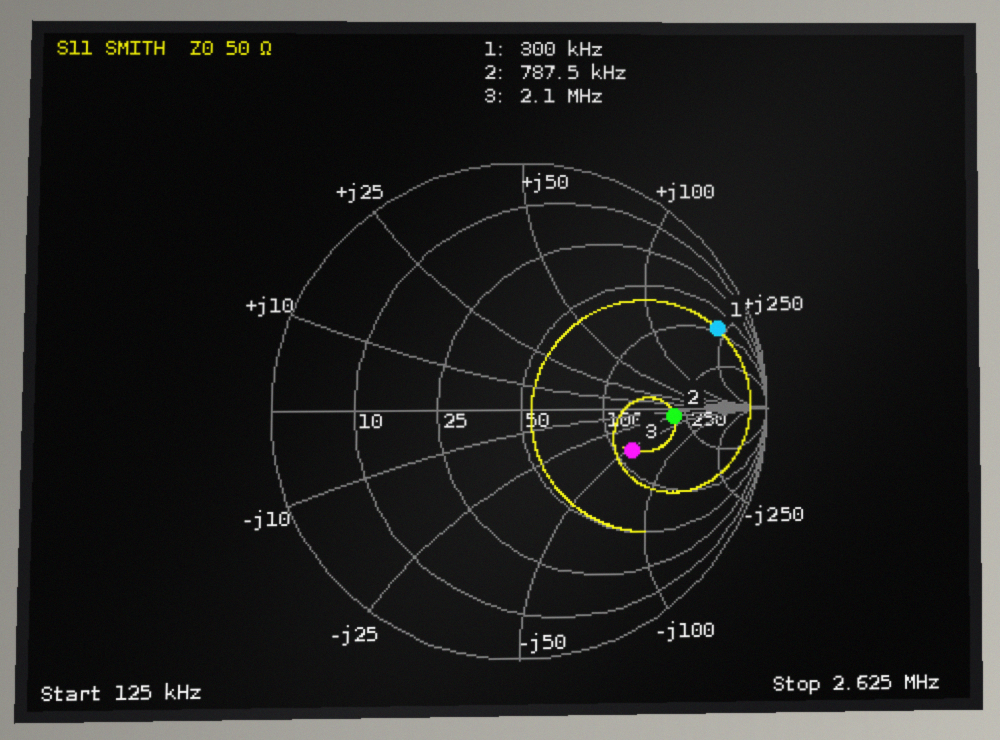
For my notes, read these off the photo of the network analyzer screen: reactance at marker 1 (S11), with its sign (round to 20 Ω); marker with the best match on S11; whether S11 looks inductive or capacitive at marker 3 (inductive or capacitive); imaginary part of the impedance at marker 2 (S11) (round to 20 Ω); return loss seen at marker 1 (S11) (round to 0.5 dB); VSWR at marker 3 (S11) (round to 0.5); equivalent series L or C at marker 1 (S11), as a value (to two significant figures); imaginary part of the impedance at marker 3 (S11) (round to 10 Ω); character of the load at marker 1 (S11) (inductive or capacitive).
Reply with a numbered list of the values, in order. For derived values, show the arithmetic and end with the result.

1. +220 Ω
2. marker 3
3. capacitive
4. -20 Ω
5. 1.5 dB
6. 3.0
7. L = 220 Ω/(2π × 300 kHz) ≈ 117 µH, so 120 µH to two significant figures
8. -50 Ω
9. inductive
